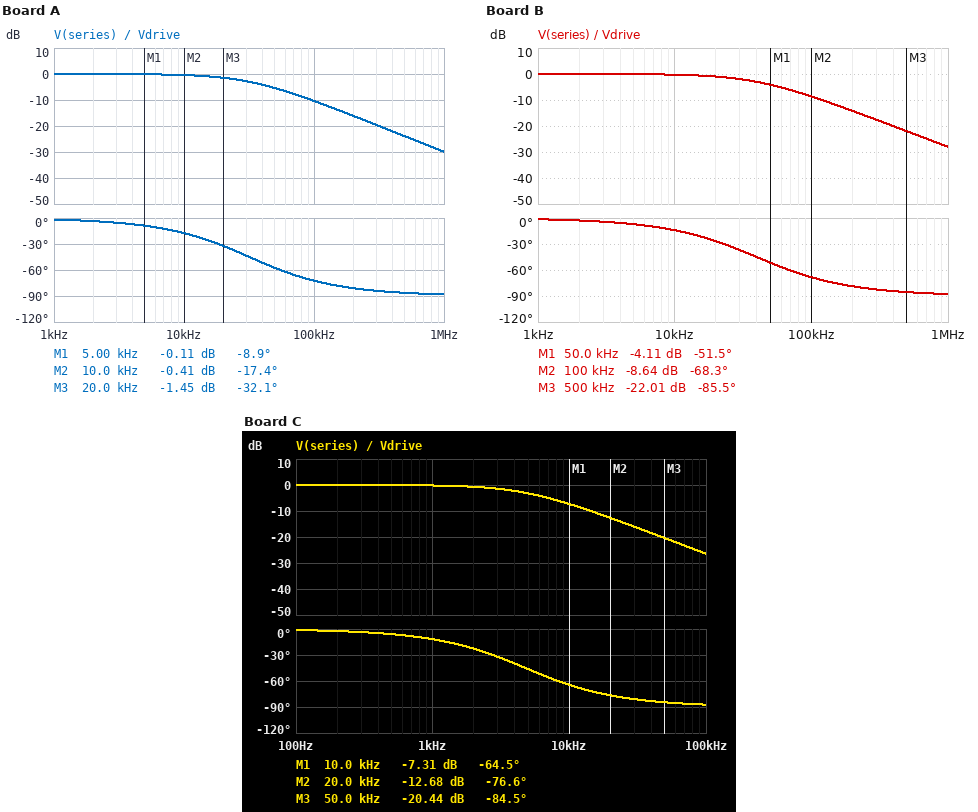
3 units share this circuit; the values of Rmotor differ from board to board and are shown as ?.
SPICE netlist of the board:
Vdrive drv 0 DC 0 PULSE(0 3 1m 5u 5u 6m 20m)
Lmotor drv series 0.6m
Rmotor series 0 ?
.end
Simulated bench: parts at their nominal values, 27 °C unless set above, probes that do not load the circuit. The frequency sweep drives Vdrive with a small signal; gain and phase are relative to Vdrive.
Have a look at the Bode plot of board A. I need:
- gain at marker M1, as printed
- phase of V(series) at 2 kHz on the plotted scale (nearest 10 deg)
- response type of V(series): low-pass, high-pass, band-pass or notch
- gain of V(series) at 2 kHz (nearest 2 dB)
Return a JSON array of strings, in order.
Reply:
["-0.11 dB", "0 deg", "low-pass", "0 dB"]
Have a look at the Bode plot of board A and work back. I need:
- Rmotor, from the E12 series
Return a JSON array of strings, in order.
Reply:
["120 Ω"]
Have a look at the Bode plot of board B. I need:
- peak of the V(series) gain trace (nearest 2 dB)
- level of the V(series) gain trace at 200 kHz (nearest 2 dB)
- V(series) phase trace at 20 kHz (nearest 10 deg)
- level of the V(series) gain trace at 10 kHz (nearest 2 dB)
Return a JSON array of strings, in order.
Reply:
["0 dB", "-14 dB", "-30 deg", "0 dB"]
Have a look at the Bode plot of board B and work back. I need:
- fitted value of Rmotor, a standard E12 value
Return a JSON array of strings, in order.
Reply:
["150 Ω"]
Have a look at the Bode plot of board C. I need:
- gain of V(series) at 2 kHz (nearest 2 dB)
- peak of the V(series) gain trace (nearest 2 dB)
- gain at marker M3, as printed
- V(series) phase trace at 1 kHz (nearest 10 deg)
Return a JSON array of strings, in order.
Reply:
["0 dB", "0 dB", "-20.44 dB", "-10 deg"]
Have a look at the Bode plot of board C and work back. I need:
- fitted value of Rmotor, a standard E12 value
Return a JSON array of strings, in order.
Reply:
["18 Ω"]
